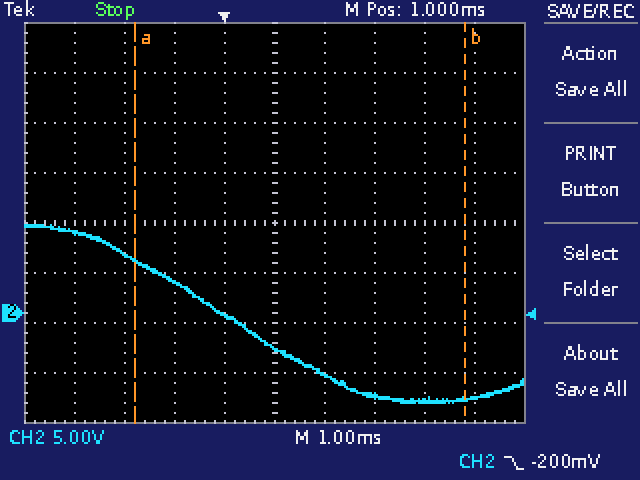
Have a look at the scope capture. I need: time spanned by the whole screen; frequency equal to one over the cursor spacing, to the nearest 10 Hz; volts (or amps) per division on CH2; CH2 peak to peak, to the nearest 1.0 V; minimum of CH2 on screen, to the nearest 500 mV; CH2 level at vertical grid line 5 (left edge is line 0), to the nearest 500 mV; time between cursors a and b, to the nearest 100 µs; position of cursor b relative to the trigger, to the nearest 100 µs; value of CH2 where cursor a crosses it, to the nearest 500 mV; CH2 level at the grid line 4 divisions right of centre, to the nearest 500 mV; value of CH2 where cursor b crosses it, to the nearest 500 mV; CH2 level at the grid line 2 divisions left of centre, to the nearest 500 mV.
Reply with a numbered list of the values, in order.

1. 10 ms
2. 150 Hz
3. 5 V
4. 18.0 V
5. -9.0 V
6. -3.5 V
7. 6.6 ms
8. +4.8 ms
9. 5.0 V
10. -8.5 V
11. -8.5 V
12. 3.0 V
